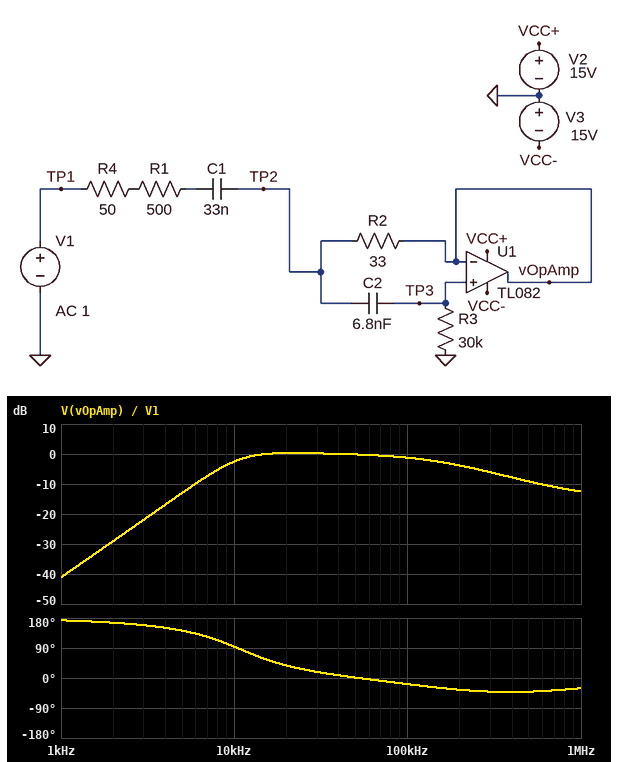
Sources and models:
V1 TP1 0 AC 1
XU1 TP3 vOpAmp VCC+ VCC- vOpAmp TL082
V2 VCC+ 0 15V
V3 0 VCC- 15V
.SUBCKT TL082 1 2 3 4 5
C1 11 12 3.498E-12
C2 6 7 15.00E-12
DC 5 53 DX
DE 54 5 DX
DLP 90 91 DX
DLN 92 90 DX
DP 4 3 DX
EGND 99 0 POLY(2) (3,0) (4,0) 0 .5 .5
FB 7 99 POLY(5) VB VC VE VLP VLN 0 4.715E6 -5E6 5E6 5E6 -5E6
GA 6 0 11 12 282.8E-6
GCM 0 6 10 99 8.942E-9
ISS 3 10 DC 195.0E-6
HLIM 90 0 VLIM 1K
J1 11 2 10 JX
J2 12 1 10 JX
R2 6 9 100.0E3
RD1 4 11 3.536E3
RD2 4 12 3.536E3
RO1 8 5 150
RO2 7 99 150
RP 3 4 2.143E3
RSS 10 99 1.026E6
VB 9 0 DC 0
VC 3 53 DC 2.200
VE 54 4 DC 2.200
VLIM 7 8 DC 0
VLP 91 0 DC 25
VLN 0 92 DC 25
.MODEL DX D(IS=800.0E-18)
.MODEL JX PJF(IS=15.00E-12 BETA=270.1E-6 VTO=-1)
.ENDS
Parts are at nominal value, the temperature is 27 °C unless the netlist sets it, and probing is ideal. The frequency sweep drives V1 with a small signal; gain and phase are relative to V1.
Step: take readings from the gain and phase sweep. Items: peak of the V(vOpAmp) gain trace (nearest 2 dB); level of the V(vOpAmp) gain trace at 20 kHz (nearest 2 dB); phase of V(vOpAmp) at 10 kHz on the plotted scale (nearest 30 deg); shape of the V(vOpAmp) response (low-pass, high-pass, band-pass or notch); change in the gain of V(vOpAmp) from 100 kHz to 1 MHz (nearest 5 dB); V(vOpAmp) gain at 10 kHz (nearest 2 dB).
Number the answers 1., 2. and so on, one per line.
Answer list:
1. 0 dB
2. 0 dB
3. 90 deg
4. band-pass
5. -10 dB
6. -2 dB
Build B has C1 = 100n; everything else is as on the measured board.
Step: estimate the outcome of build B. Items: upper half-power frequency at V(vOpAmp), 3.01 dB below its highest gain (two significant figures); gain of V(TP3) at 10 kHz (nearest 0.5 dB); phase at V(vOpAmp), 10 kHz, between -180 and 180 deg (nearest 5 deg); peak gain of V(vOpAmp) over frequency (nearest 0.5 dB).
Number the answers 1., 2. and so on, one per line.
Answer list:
1. 180 kHz
2. -3.5 dB
3. 65 deg
4. 0 dB
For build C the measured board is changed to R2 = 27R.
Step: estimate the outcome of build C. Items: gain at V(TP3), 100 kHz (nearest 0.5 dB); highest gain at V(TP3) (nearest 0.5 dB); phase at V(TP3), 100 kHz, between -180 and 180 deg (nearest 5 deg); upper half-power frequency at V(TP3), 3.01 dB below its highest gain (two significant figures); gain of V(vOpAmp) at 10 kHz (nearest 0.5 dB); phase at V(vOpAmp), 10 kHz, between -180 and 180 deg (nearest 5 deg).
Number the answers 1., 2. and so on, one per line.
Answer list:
1. -1.5 dB
2. 0 dB
3. -20 deg
4. 140 kHz
5. -4.5 dB
6. 100 deg
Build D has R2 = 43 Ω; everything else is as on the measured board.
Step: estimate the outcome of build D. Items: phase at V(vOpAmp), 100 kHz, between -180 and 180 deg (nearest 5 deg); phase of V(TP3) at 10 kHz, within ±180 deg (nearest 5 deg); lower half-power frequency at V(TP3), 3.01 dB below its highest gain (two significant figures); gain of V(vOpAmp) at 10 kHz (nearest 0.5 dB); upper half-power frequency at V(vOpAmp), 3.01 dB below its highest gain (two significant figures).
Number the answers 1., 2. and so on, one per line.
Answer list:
1. -15 deg
2. 80 deg
3. 8.2 kHz
4. -0.5 dB
5. 180 kHz
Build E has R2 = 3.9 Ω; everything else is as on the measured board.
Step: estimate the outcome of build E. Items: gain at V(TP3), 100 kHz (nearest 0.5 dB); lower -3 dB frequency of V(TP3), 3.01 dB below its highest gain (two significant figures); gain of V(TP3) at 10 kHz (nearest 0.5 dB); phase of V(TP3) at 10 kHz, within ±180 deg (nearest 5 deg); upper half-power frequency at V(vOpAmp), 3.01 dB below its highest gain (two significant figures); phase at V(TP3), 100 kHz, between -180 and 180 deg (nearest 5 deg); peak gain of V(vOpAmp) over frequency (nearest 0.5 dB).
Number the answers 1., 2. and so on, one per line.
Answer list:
1. -9.0 dB
2. 37 kHz
3. -22.5 dB
4. 135 deg
5. 55 kHz
6. -25 deg
7. 1.5 dB
